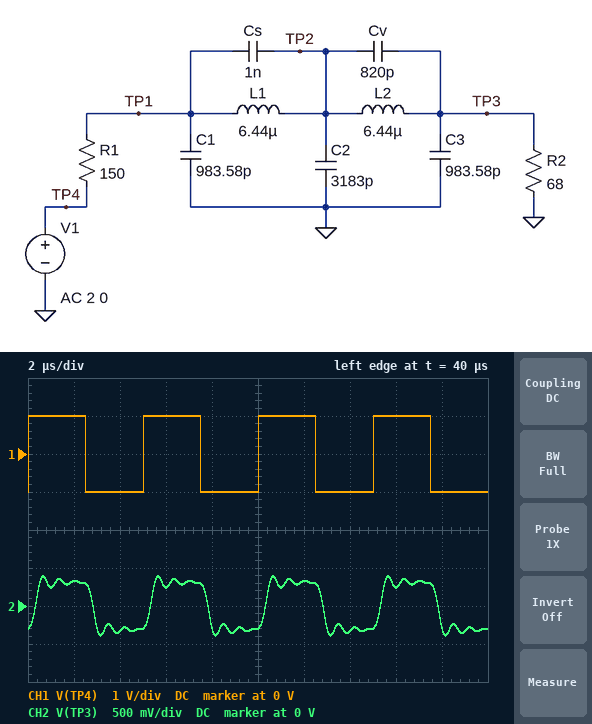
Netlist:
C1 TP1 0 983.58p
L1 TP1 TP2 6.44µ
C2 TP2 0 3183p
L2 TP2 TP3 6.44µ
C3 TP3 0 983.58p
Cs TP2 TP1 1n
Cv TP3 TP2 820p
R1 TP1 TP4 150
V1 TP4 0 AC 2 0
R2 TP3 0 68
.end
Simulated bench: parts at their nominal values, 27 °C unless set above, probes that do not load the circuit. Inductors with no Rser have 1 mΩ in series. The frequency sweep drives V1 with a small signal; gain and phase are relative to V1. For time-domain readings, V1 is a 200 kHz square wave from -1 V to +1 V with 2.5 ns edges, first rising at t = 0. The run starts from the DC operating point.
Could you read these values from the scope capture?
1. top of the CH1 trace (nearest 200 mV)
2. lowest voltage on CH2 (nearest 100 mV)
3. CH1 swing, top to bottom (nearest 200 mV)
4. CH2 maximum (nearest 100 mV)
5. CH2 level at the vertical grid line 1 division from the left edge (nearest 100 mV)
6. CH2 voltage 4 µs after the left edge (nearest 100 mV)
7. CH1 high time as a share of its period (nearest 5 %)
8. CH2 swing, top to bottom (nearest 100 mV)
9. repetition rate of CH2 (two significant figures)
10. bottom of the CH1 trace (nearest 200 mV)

1.0 V
-400 mV
2.0 V
400 mV
300 mV
-300 mV
50 %
800 mV
200 kHz
-1.0 V
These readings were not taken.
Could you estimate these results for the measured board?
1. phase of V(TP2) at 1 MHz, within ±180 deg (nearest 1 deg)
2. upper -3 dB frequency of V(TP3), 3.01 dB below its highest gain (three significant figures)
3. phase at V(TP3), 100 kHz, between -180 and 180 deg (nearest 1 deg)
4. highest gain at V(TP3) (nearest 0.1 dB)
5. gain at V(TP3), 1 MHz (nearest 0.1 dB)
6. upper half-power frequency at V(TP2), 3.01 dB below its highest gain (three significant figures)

-61 deg
1.52 MHz
-11 deg
-10.1 dB
-11.0 dB
1.57 MHz
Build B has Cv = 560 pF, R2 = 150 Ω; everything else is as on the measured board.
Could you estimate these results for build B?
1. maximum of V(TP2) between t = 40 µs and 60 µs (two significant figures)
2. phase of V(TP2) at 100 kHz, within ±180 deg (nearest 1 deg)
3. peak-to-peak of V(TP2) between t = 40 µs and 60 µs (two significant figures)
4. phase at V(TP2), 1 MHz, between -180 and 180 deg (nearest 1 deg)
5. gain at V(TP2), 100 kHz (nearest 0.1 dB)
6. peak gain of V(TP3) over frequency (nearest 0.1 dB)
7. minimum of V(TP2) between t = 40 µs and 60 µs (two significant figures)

500 mV
-14 deg
1.0 V
-78 deg
-6.2 dB
-6.0 dB
-500 mV
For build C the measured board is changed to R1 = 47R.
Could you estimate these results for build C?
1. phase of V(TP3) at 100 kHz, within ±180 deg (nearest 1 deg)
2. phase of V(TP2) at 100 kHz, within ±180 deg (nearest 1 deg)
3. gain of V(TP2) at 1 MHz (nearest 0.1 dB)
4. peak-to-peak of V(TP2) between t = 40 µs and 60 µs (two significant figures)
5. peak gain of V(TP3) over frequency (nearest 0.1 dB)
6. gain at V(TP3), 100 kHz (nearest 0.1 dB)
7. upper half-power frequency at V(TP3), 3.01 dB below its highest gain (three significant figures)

-9 deg
-6 deg
-4.3 dB
1.6 V
-4.4 dB
-4.6 dB
1.40 MHz
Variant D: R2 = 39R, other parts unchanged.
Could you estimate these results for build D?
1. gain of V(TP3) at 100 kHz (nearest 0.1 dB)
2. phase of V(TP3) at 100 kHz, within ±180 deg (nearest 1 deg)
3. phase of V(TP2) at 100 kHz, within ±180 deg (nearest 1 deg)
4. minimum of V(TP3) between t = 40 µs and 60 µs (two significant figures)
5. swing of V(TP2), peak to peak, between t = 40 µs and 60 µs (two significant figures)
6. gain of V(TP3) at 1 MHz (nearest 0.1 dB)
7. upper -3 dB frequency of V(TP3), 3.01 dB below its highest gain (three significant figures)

-13.7 dB
-8 deg
-2 deg
-310 mV
810 mV
-12.5 dB
1.47 MHz
